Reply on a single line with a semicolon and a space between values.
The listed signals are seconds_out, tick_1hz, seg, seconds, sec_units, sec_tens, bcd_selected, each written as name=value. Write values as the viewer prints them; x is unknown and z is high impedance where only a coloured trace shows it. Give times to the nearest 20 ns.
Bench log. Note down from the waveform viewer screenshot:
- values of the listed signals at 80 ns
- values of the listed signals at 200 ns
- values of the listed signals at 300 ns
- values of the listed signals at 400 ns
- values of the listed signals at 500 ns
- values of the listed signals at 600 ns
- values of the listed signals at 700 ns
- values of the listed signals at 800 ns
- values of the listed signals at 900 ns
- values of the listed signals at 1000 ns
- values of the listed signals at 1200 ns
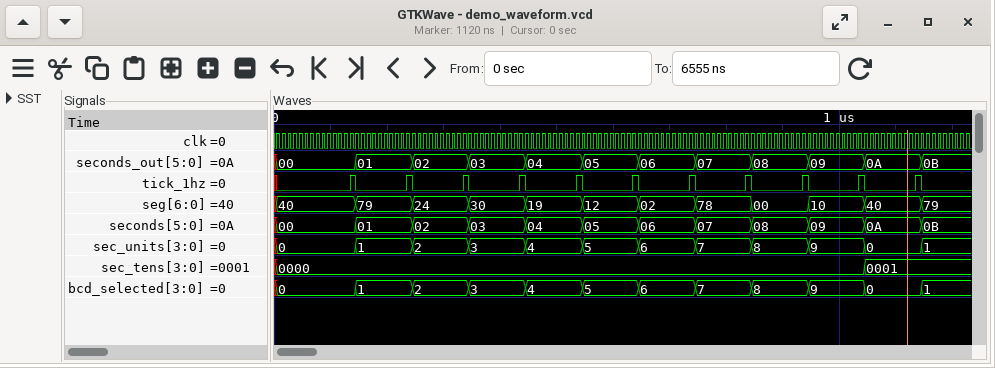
seconds_out=00, tick_1hz=0, seg=40, seconds=00, sec_units=0, sec_tens=0000, bcd_selected=0; seconds_out=01, tick_1hz=0, seg=79, seconds=01, sec_units=1, sec_tens=0000, bcd_selected=1; seconds_out=02, tick_1hz=0, seg=24, seconds=02, sec_units=2, sec_tens=0000, bcd_selected=2; seconds_out=03, tick_1hz=0, seg=30, seconds=03, sec_units=3, sec_tens=0000, bcd_selected=3; seconds_out=04, tick_1hz=0, seg=19, seconds=04, sec_units=4, sec_tens=0000, bcd_selected=4; seconds_out=05, tick_1hz=0, seg=12, seconds=05, sec_units=5, sec_tens=0000, bcd_selected=5; seconds_out=06, tick_1hz=0, seg=02, seconds=06, sec_units=6, sec_tens=0000, bcd_selected=6; seconds_out=07, tick_1hz=0, seg=78, seconds=07, sec_units=7, sec_tens=0000, bcd_selected=7; seconds_out=08, tick_1hz=0, seg=00, seconds=08, sec_units=8, sec_tens=0000, bcd_selected=8; seconds_out=09, tick_1hz=0, seg=10, seconds=09, sec_units=9, sec_tens=0000, bcd_selected=9; seconds_out=0B, tick_1hz=0, seg=79, seconds=0B, sec_units=1, sec_tens=0001, bcd_selected=1
